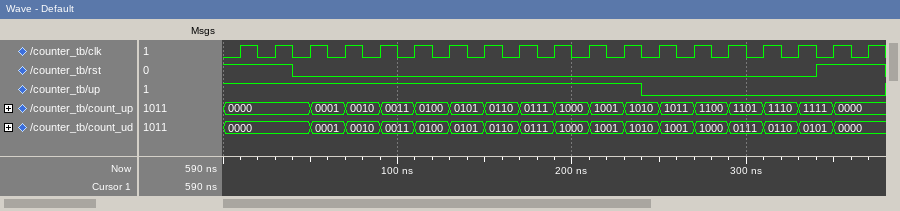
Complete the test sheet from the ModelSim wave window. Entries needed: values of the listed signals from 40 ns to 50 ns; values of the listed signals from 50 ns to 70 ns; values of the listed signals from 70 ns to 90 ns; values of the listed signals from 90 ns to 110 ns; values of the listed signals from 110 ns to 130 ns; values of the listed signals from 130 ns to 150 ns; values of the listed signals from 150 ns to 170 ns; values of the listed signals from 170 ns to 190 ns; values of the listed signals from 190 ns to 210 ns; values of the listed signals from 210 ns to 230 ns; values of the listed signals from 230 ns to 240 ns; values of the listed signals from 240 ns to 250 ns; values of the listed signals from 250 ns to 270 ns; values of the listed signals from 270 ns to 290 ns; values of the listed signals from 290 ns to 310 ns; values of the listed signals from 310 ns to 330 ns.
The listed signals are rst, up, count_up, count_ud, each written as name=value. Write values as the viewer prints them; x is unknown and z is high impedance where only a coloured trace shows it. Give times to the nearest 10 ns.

rst=0, up=1, count_up=0000, count_ud=0000
rst=0, up=1, count_up=0001, count_ud=0001
rst=0, up=1, count_up=0010, count_ud=0010
rst=0, up=1, count_up=0011, count_ud=0011
rst=0, up=1, count_up=0100, count_ud=0100
rst=0, up=1, count_up=0101, count_ud=0101
rst=0, up=1, count_up=0110, count_ud=0110
rst=0, up=1, count_up=0111, count_ud=0111
rst=0, up=1, count_up=1000, count_ud=1000
rst=0, up=1, count_up=1001, count_ud=1001
rst=0, up=1, count_up=1010, count_ud=1010
rst=0, up=0, count_up=1010, count_ud=1010
rst=0, up=0, count_up=1011, count_ud=1001
rst=0, up=0, count_up=1100, count_ud=1000
rst=0, up=0, count_up=1101, count_ud=0111
rst=0, up=0, count_up=1110, count_ud=0110
